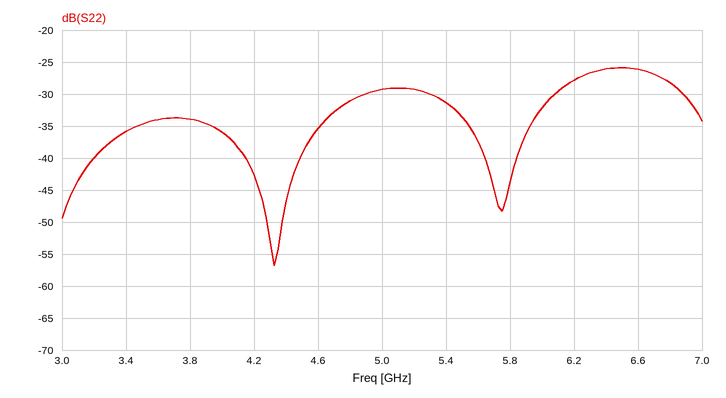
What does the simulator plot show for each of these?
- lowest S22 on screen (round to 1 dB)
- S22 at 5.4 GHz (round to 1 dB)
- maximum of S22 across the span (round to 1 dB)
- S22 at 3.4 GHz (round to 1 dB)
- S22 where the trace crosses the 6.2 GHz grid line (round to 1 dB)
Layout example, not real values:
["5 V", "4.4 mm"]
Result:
["-57 dB", "-31 dB", "-26 dB", "-36 dB", "-28 dB"]
